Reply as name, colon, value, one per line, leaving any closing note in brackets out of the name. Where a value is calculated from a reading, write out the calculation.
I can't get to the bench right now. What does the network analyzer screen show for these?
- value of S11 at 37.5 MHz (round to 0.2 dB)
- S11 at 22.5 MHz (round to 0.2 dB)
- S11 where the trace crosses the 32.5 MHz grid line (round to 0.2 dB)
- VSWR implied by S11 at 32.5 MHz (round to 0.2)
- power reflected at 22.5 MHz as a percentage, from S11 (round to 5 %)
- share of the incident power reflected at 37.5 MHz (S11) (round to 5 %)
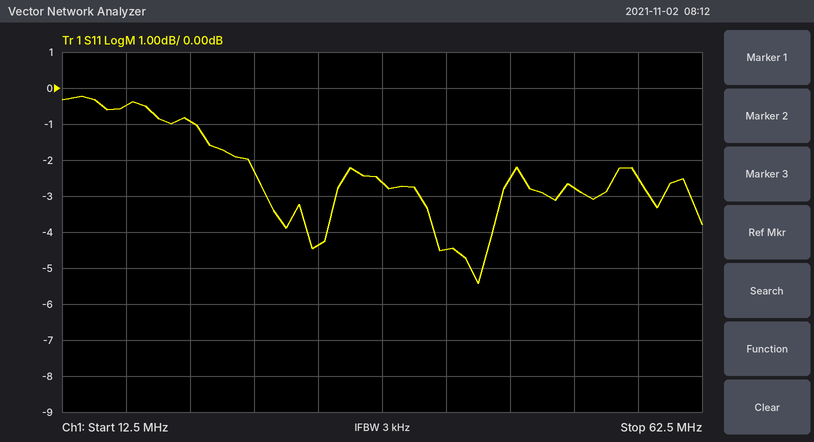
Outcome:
value of S11 at 37.5 MHz: -2.6 dB
S11 at 22.5 MHz: -1.0 dB
S11 where the trace crosses the 32.5 MHz grid line: -4.4 dB
VSWR implied by S11 at 32.5 MHz: |Γ| = 10^(-4.4/20) = 0.6026; VSWR = (1 + 0.6026)/(1 − 0.6026) ≈ 4.0
power reflected at 22.5 MHz as a percentage, from S11: 10^(-1/10) ≈ 79.4 %, so 80 % to the nearest 5 %
share of the incident power reflected at 37.5 MHz (S11): 10^(-2.6/10) ≈ 55 %
